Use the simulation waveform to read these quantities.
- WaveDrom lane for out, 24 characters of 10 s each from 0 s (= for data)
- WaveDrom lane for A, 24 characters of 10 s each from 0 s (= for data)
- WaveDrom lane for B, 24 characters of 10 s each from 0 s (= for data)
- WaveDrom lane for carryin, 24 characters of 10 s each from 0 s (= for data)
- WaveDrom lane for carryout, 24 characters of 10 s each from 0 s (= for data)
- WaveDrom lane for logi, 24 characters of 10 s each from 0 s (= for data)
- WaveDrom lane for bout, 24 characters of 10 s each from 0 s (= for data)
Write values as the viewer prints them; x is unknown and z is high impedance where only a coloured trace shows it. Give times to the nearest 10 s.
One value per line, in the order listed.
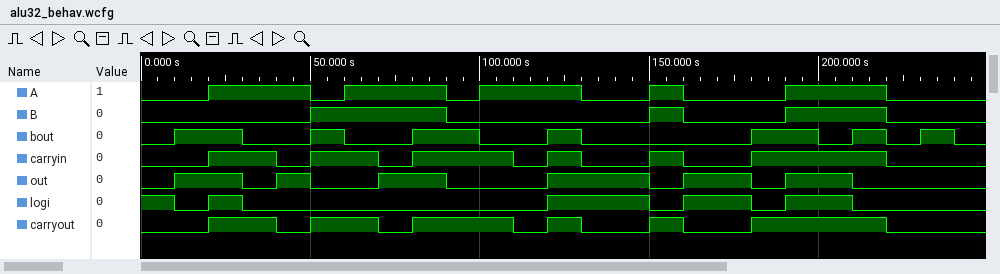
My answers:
{name: 'out', wave: '01.010.1.0..1..01.01.0..'}
{name: 'A', wave: '0.1..01..01..0.10..1..0.'}
{name: 'B', wave: '0....1...0.....10..1..0.'}
{name: 'carryin', wave: '0.1.01.01..010.10.1...0.'}
{name: 'carryout', wave: '0.1.01.01..010.10.1...0.'}
{name: 'logi', wave: '1010........1..01.01.0..'}
{name: 'bout', wave: '01.0.10.1.0.10....1.0101'}
